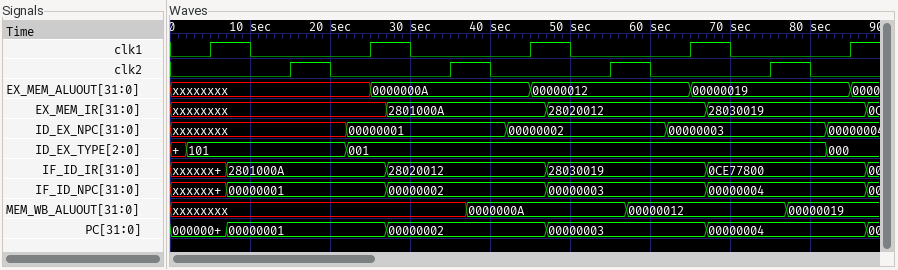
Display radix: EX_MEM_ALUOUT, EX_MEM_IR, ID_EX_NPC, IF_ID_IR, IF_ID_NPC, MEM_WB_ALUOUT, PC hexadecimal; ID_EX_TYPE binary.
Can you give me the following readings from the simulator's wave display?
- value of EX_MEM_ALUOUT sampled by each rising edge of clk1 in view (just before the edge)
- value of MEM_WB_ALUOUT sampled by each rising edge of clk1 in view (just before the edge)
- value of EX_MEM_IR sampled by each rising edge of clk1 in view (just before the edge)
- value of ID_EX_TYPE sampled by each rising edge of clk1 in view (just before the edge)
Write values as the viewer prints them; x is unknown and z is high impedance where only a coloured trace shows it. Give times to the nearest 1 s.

xxxxxxxx, xxxxxxxx, 0000000A, 00000012, 00000019
xxxxxxxx, xxxxxxxx, 0000000A, 00000012, 00000019
xxxxxxxx, xxxxxxxx, 2801000A, 28020012, 28030019
101, 001, 001, 001, 000
